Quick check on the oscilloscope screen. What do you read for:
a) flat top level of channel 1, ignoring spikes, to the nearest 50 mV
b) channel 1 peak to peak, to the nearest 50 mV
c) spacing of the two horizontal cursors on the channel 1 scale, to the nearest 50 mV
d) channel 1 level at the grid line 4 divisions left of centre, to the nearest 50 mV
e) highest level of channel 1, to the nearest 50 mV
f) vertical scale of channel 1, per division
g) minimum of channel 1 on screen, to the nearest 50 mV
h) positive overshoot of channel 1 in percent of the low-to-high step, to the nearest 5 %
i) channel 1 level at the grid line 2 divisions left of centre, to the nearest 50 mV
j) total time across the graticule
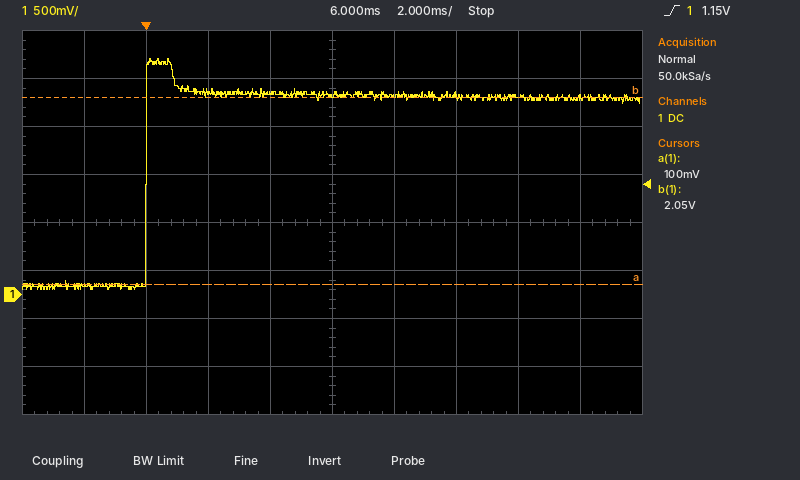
2.05 V
2.40 V
1.95 V
100 mV
2.45 V
500 mV
50 mV
20 %
2.10 V
20 ms
